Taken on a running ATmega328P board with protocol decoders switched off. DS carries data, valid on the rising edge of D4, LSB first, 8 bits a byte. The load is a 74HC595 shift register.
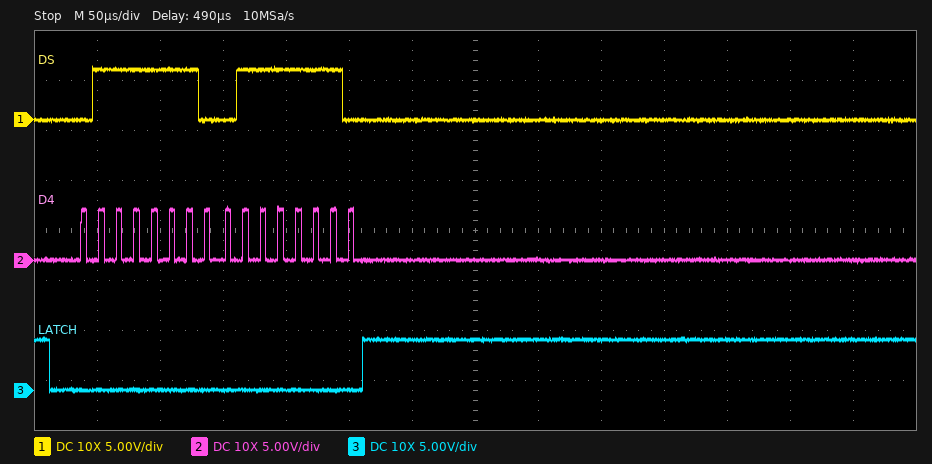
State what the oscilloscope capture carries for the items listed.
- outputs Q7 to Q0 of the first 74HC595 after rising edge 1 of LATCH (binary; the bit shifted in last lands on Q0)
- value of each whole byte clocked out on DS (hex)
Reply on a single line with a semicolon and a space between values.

01111110; 7E 7E
